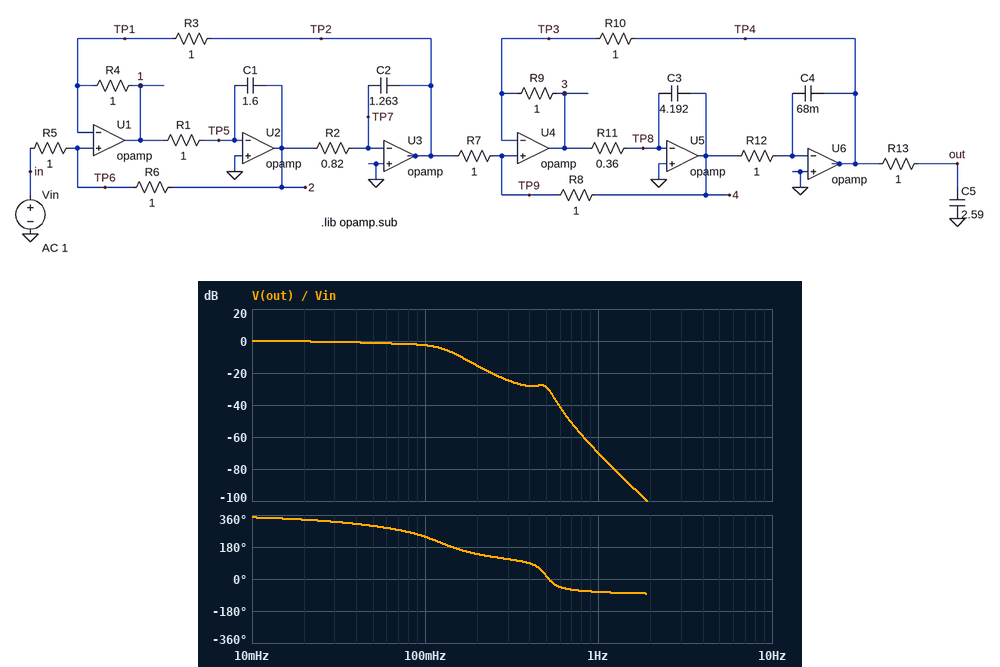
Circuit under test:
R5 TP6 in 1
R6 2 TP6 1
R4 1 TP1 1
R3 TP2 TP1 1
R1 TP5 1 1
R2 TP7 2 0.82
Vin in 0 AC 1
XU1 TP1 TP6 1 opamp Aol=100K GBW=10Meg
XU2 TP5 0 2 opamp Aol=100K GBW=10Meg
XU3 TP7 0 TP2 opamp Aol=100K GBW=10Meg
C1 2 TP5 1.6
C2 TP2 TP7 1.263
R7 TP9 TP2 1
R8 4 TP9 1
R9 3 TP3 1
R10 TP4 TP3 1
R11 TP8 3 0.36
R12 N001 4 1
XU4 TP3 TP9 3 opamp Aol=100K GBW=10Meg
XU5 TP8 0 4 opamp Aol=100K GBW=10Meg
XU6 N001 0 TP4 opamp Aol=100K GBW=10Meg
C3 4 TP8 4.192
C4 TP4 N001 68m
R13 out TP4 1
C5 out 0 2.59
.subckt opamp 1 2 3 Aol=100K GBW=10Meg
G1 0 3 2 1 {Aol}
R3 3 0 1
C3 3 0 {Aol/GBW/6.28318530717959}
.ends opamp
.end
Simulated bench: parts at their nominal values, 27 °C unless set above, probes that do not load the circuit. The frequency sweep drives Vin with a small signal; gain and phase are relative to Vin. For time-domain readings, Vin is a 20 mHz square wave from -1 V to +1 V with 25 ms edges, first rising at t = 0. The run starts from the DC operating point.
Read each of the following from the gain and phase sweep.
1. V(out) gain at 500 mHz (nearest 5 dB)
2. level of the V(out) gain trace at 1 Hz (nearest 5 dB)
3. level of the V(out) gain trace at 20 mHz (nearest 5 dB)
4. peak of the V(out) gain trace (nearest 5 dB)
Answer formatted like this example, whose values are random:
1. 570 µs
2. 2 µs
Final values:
1. -30 dB
2. -70 dB
3. 0 dB
4. 0 dB
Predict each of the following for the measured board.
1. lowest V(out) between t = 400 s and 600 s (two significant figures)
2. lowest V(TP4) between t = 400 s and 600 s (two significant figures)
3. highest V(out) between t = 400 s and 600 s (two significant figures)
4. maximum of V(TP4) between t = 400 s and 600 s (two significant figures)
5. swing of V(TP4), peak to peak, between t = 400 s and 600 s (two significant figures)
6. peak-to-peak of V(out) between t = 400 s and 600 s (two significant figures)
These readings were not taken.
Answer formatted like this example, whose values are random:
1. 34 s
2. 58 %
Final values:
1. -1.0 V
2. -1.6 V
3. 1.0 V
4. 1.6 V
5. 3.1 V
6. 2.0 V
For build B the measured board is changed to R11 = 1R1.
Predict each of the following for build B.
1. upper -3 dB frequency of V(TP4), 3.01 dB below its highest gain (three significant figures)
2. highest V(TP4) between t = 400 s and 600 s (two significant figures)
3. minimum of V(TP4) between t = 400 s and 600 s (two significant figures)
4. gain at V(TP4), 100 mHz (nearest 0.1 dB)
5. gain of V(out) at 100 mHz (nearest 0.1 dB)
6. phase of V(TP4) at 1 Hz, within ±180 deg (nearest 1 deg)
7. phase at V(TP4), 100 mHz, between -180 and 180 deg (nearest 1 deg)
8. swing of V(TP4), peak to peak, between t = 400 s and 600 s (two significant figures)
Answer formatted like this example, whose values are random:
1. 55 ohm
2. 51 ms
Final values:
1. 296 mHz
2. 1.8 V
3. -1.8 V
4. 3.8 dB
5. -1.8 dB
6. 8 deg
7. -65 deg
8. 3.6 V
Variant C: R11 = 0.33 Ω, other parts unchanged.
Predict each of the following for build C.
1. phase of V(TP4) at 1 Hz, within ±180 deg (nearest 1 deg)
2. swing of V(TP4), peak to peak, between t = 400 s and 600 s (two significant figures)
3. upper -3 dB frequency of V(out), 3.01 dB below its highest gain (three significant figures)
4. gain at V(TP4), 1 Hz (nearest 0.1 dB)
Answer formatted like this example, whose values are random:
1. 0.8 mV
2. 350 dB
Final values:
1. 15 deg
2. 3.1 V
3. 106 mHz
4. -45.0 dB
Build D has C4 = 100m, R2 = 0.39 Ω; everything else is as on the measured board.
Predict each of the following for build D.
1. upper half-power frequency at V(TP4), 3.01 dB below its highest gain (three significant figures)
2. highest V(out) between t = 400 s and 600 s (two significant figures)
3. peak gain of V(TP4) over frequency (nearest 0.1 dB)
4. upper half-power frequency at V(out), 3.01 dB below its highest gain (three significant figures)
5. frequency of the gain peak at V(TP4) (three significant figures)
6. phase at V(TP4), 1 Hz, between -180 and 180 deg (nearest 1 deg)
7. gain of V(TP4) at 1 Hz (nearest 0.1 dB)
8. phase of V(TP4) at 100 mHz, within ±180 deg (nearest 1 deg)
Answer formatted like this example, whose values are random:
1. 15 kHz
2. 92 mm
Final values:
1. 223 mHz
2. 1.0 V
3. 7.0 dB
4. 181 mHz
5. 171 mHz
6. 13 deg
7. -43.6 dB
8. -28 deg
